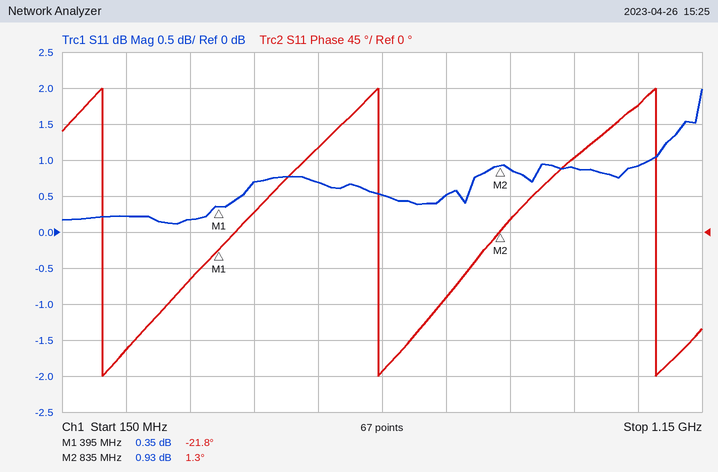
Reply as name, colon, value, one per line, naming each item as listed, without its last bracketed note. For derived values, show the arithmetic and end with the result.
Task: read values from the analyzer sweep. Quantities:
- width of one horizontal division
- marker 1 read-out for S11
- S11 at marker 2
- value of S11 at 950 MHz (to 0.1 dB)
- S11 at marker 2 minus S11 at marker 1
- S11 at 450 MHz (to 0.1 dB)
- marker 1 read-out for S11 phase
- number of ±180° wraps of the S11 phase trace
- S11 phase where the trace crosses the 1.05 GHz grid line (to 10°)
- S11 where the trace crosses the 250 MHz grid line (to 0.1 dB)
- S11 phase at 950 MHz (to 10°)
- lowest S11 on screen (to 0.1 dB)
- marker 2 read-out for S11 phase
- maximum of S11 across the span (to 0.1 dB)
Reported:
width of one horizontal division: 100 MHz
marker 1 read-out for S11: 0.35 dB
S11 at marker 2: 0.93 dB
value of S11 at 950 MHz: 0.9 dB
S11 at marker 2 minus S11 at marker 1: 0.93 − (0.35) = 0.58 dB
S11 at 450 MHz: 0.7 dB
marker 1 read-out for S11 phase: -21.8°
number of ±180° wraps of the S11 phase trace: 3
S11 phase where the trace crosses the 1.05 GHz grid line: 160°
S11 where the trace crosses the 250 MHz grid line: 0.2 dB
S11 phase at 950 MHz: 90°
lowest S11 on screen: 0.1 dB
marker 2 read-out for S11 phase: 1.3°
maximum of S11 across the span: 2.0 dB
